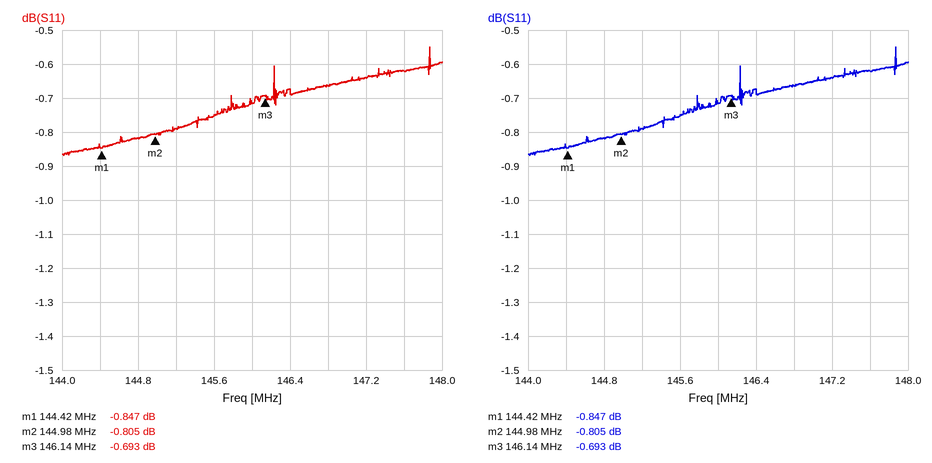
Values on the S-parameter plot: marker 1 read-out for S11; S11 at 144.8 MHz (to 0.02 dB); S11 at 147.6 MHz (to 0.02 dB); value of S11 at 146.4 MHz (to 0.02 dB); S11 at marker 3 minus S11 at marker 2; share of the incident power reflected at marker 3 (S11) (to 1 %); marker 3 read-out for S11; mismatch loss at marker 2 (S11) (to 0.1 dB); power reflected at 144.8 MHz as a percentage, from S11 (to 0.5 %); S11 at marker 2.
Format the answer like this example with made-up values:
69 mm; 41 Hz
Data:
-0.847 dB; -0.82 dB; -0.62 dB; -0.68 dB; 0.112 dB; 85 %; -0.693 dB; 7.7 dB; 83.0 %; -0.805 dB
